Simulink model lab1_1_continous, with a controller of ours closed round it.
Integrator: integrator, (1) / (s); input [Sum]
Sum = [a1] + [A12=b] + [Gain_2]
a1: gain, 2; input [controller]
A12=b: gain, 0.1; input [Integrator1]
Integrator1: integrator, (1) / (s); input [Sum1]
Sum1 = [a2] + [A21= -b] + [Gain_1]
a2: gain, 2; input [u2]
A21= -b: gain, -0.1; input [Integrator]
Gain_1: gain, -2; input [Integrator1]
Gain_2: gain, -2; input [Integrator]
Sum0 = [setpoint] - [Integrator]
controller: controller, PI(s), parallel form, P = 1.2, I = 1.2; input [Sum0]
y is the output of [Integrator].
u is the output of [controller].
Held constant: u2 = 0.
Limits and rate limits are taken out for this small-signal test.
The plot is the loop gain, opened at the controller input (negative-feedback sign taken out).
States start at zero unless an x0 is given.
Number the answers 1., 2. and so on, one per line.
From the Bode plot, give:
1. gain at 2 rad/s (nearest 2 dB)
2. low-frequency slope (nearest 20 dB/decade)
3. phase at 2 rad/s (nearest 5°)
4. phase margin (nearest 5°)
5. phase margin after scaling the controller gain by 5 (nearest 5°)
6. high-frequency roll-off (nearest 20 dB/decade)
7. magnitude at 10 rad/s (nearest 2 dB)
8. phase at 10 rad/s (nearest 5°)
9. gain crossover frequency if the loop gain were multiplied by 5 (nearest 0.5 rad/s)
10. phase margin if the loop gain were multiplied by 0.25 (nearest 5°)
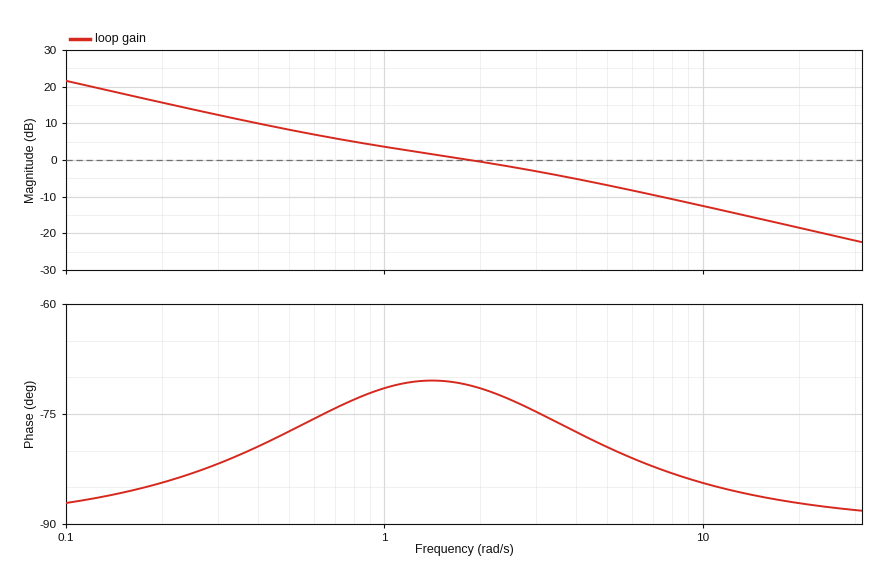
1. 0 dB
2. -20 dB/decade
3. -70°
4. 110°
5. 95°
6. -20 dB/decade
7. -12 dB
8. -85°
9. 12.0 rad/s
10. 100°
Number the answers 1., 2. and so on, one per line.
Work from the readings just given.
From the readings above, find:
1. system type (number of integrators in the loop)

1. 1
